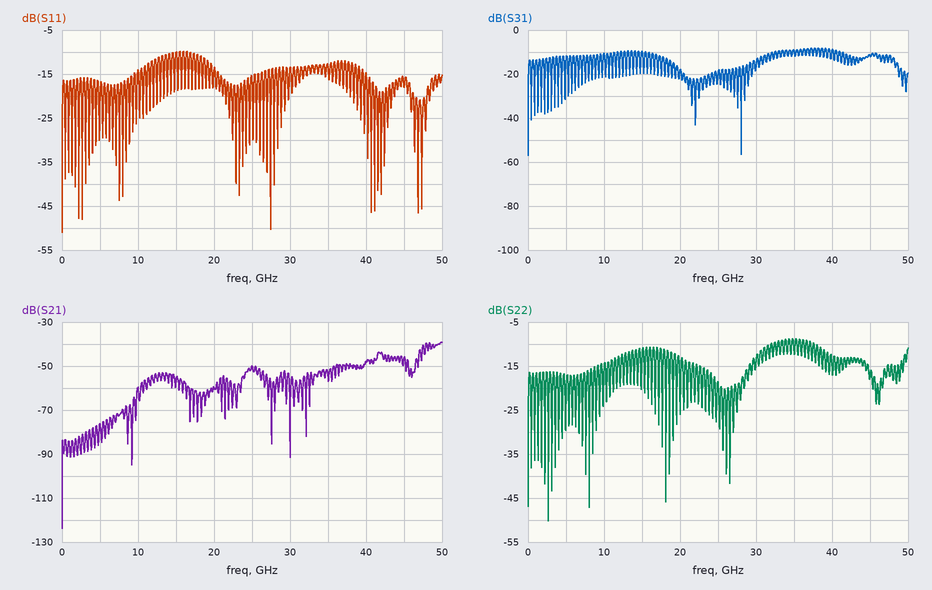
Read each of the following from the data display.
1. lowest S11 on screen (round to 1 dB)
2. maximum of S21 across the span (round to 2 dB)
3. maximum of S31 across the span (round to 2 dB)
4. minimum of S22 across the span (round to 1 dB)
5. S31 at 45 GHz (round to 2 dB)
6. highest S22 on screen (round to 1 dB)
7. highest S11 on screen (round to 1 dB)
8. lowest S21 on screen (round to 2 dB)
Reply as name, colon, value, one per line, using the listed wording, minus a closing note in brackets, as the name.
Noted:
lowest S11 on screen: -51 dB
maximum of S21 across the span: -40 dB
maximum of S31 across the span: -8 dB
minimum of S22 across the span: -50 dB
S31 at 45 GHz: -12 dB
highest S22 on screen: -9 dB
highest S11 on screen: -10 dB
lowest S21 on screen: -124 dB
